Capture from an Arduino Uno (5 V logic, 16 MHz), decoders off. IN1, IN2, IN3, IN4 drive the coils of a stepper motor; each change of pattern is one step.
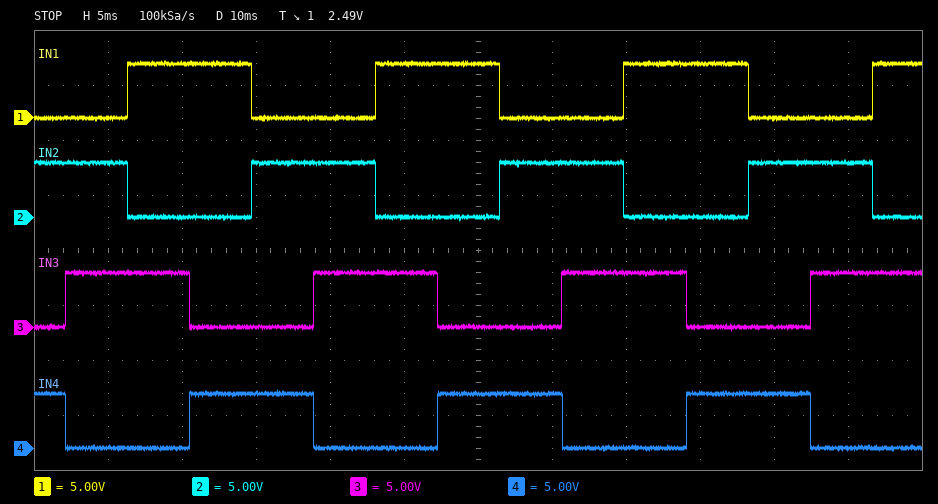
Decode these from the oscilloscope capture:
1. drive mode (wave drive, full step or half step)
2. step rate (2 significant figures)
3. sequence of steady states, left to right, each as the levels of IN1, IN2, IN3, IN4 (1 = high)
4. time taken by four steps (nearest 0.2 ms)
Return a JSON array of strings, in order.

["full step", "240 steps/s", "0101 0110 1010 1001 0101 0110 1010 1001 0101 0110 1010 1001 0101 0110 1010", "16.8 ms"]
